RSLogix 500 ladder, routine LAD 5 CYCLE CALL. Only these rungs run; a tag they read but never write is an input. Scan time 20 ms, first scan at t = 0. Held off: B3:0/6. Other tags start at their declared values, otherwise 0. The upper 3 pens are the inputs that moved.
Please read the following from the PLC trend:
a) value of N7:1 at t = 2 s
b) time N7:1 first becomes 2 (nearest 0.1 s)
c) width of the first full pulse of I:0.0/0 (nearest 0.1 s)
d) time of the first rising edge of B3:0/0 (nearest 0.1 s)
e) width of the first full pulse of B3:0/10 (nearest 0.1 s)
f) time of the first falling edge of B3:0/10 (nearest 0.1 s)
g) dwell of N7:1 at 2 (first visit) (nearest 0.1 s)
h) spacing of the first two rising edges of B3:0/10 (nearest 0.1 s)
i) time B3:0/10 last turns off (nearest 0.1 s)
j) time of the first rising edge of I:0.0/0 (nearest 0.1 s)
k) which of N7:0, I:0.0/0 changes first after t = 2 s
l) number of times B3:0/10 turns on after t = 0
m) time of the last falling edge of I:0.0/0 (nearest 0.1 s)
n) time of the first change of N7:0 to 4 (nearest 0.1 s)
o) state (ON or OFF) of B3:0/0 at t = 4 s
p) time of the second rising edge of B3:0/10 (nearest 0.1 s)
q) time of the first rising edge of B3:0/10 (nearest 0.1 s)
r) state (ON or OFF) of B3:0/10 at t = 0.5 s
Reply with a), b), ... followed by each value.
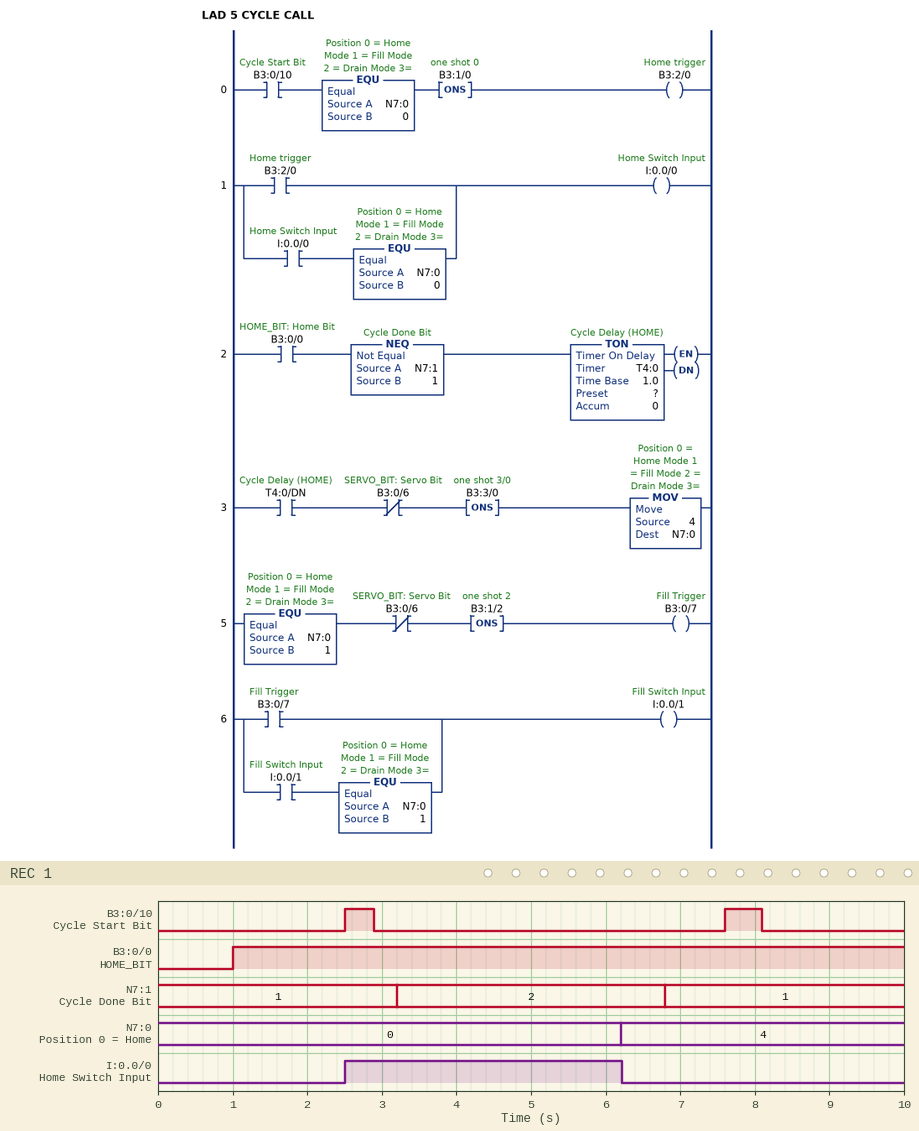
a) 1
b) 3.2 s
c) 3.7 s
d) 1.0 s
e) 0.4 s
f) 2.9 s
g) 3.6 s
h) 5.1 s
i) 8.1 s
j) 2.5 s
k) I:0.0/0
l) 2
m) 6.2 s
n) 6.2 s
o) ON
p) 7.6 s
q) 2.5 s
r) OFF
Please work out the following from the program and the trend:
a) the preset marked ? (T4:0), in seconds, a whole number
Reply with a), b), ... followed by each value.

a) 3 s
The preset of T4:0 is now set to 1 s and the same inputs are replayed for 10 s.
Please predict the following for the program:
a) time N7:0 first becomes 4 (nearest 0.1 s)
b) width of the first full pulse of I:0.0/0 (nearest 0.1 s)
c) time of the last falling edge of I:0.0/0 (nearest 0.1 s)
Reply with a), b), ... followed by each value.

a) 4.2 s
b) 1.7 s
c) 4.2 s
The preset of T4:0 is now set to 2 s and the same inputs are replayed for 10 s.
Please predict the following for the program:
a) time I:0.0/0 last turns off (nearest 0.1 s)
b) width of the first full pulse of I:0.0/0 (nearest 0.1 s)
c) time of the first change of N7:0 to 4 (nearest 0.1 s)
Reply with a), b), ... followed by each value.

a) 5.2 s
b) 2.7 s
c) 5.2 s
